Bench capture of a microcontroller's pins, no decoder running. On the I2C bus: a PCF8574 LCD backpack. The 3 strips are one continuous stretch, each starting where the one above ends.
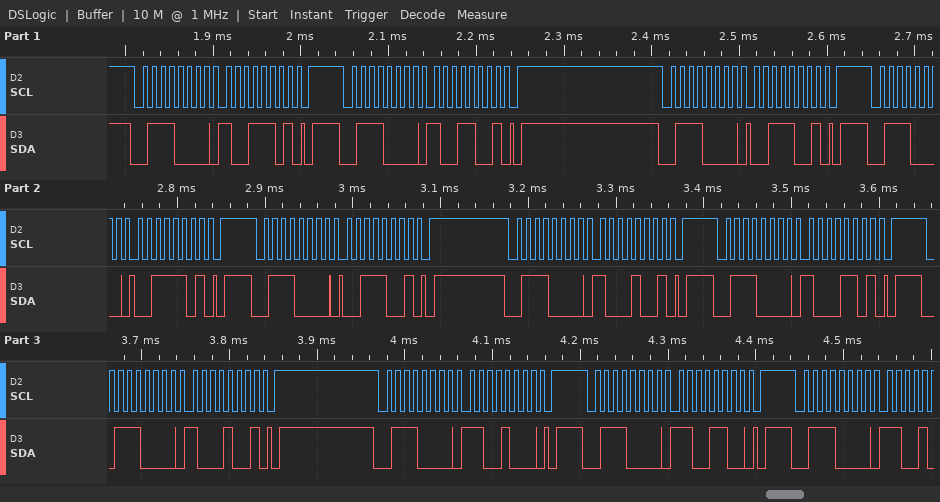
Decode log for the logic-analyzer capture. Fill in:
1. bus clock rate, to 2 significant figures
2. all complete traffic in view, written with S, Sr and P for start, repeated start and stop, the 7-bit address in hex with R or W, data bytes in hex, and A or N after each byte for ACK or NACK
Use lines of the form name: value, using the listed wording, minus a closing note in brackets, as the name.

bus clock rate, to 2 significant figures: 100 kHz
all complete traffic in view, written with S, Sr and P for start, repeated start and stop, the 7-bit address in hex with R or W, data bytes in hex, and A or N after each byte for ACK or NACK: S 38W A 9D A P S 38W A 99 A P S 38W A 39 A P S 38W A 3D A P S 38W A 39 A P S 38W A 89 A P S 38W A 8D A P S 38W A 89 A P S 38W A C8 A P S 38W A CC A P S 38W A
